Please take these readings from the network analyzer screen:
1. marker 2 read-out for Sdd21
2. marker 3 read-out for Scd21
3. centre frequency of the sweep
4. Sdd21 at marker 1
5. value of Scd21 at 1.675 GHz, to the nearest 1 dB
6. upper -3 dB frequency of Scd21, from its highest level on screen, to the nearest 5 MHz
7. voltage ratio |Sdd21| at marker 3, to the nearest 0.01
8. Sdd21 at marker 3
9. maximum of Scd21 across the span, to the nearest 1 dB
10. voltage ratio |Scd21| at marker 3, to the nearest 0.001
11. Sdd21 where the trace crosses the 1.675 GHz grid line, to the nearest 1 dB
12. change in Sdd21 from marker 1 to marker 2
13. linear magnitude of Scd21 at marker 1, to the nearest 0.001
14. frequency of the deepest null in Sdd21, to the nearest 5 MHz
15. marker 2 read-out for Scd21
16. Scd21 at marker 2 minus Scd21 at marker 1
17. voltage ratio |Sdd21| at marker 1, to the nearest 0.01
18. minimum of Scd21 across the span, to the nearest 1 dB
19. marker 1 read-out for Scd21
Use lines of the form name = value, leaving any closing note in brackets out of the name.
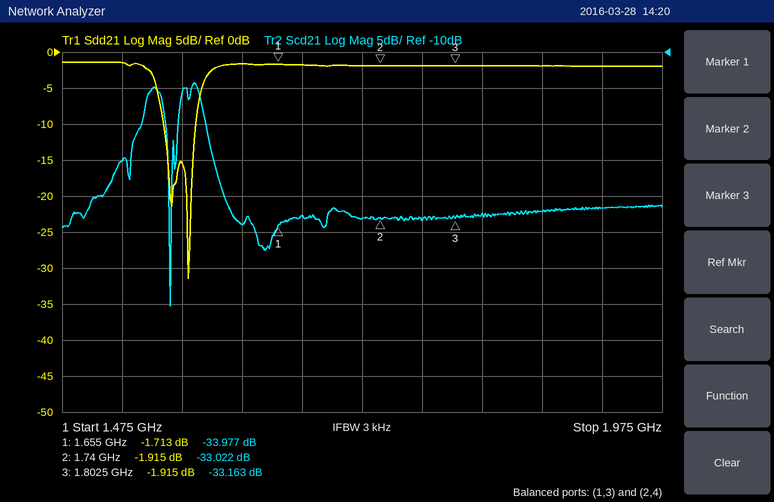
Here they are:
marker 2 read-out for Sdd21 = -1.915 dB
marker 3 read-out for Scd21 = -33.163 dB
centre frequency of the sweep = 1.725 GHz
Sdd21 at marker 1 = -1.713 dB
value of Scd21 at 1.675 GHz, to the nearest 1 dB = -33 dB
upper -3 dB frequency of Scd21, from its highest level on screen, to the nearest 5 MHz = 1.590 GHz
voltage ratio |Sdd21| at marker 3, to the nearest 0.01 = 0.80
Sdd21 at marker 3 = -1.915 dB
maximum of Scd21 across the span, to the nearest 1 dB = -14 dB
voltage ratio |Scd21| at marker 3, to the nearest 0.001 = 0.022
Sdd21 where the trace crosses the 1.675 GHz grid line, to the nearest 1 dB = -2 dB
change in Sdd21 from marker 1 to marker 2 = -0.202 dB
linear magnitude of Scd21 at marker 1, to the nearest 0.001 = 0.020
frequency of the deepest null in Sdd21, to the nearest 5 MHz = 1.580 GHz
marker 2 read-out for Scd21 = -33.022 dB
Scd21 at marker 2 minus Scd21 at marker 1 = 0.955 dB
voltage ratio |Sdd21| at marker 1, to the nearest 0.01 = 0.82
minimum of Scd21 across the span, to the nearest 1 dB = -45 dB
marker 1 read-out for Scd21 = -33.977 dB
